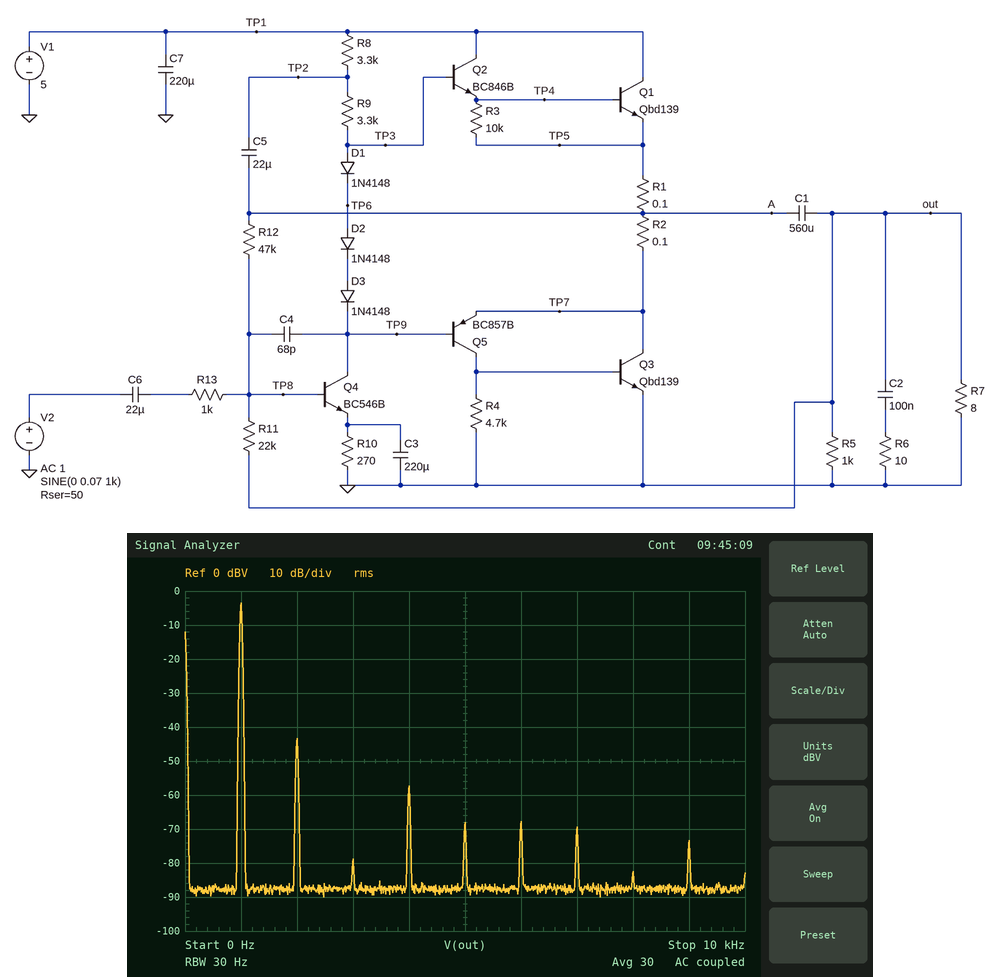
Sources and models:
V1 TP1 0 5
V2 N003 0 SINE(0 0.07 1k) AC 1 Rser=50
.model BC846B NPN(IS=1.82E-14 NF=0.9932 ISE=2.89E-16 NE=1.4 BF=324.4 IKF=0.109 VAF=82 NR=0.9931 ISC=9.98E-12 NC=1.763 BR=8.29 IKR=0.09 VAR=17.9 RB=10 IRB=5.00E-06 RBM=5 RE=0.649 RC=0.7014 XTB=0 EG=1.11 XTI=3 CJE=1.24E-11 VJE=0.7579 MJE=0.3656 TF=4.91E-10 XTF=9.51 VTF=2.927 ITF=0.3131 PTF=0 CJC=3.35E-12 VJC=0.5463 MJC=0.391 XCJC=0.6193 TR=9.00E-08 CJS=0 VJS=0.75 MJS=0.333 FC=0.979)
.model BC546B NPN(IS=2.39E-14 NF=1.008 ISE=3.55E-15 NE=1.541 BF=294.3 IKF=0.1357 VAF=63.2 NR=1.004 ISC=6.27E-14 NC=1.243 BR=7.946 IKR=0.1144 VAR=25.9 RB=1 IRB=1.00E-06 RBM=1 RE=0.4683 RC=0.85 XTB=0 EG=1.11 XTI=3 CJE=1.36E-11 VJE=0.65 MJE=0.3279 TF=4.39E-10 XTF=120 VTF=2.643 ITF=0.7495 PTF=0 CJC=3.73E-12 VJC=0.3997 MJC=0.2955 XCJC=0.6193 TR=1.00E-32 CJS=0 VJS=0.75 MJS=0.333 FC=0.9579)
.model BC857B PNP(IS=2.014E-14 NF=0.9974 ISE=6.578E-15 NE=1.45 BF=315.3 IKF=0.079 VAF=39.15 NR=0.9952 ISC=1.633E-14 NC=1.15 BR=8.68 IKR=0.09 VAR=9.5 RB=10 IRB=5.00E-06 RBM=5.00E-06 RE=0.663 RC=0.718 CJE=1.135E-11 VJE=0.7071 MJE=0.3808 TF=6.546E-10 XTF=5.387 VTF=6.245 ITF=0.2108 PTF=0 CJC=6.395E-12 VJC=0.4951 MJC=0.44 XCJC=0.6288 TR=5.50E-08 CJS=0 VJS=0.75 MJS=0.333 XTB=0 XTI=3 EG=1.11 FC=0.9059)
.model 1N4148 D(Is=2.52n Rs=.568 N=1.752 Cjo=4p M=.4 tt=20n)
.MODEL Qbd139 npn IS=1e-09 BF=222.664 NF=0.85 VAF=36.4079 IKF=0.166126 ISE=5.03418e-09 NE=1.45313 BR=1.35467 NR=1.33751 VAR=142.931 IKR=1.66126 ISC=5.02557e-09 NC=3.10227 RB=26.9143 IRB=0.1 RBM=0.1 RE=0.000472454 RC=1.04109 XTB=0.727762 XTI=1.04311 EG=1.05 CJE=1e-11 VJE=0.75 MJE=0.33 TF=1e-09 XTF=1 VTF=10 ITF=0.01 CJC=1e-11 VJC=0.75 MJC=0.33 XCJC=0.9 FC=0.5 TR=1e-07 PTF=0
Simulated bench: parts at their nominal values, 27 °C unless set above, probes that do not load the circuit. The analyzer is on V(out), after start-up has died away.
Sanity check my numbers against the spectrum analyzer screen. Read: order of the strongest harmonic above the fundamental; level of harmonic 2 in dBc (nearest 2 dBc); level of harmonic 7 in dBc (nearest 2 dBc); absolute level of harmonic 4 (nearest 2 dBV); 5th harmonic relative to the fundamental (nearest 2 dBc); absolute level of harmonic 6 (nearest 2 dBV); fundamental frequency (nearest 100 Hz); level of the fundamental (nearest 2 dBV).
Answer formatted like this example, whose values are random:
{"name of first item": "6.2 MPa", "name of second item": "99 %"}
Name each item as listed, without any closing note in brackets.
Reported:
{"order of the strongest harmonic above the fundamental": "2", "level of harmonic 2 in dBc": "-40 dBc", "level of harmonic 7 in dBc": "-66 dBc", "absolute level of harmonic 4": "-58 dBV", "5th harmonic relative to the fundamental": "-64 dBc", "absolute level of harmonic 6": "-68 dBV", "fundamental frequency": "1.0 kHz", "level of the fundamental": "-4 dBV"}
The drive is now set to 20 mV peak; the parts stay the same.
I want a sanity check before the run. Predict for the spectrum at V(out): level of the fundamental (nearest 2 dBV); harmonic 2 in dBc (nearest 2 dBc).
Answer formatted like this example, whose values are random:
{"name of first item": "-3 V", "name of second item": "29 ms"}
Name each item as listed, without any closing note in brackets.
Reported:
{"level of the fundamental": "-14 dBV", "harmonic 2 in dBc": "-46 dBc"}
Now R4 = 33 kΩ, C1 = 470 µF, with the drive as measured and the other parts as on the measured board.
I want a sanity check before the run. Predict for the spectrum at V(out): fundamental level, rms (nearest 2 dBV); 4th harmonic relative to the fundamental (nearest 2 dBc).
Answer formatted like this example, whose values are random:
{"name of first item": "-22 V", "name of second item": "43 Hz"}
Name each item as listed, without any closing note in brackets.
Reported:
{"fundamental level, rms": "-4 dBV", "4th harmonic relative to the fundamental": "-56 dBc"}
